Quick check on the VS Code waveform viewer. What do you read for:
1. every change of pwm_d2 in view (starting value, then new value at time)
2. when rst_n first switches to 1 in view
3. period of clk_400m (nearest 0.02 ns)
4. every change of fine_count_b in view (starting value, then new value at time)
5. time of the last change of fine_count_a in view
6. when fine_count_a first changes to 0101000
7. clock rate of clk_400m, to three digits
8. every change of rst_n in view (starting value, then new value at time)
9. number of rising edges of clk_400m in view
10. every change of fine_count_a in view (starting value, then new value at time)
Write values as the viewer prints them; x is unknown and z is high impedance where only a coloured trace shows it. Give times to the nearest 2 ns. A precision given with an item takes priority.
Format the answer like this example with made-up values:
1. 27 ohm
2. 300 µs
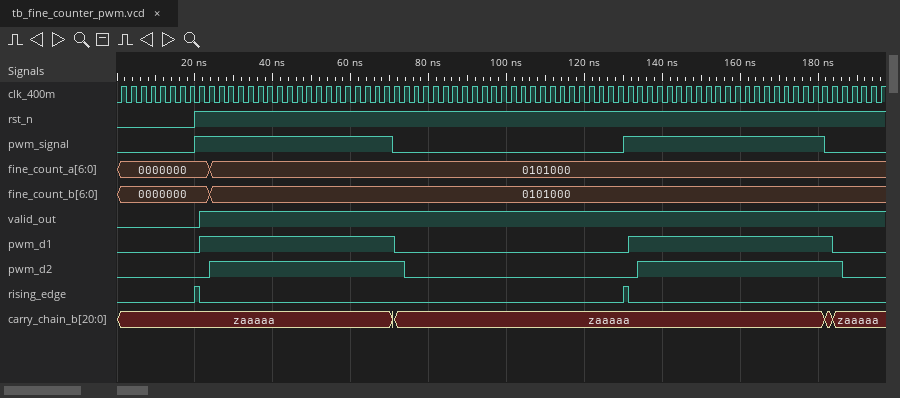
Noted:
1. 0, 1 at 24 ns, 0 at 74 ns, 1 at 134 ns, 0 at 186 ns
2. 20 ns
3. 2.5 ns
4. 0000000, 0101000 at 24 ns
5. 24 ns
6. 24 ns
7. 400 MHz
8. 0, 1 at 20 ns
9. 79
10. 0000000, 0101000 at 24 ns
